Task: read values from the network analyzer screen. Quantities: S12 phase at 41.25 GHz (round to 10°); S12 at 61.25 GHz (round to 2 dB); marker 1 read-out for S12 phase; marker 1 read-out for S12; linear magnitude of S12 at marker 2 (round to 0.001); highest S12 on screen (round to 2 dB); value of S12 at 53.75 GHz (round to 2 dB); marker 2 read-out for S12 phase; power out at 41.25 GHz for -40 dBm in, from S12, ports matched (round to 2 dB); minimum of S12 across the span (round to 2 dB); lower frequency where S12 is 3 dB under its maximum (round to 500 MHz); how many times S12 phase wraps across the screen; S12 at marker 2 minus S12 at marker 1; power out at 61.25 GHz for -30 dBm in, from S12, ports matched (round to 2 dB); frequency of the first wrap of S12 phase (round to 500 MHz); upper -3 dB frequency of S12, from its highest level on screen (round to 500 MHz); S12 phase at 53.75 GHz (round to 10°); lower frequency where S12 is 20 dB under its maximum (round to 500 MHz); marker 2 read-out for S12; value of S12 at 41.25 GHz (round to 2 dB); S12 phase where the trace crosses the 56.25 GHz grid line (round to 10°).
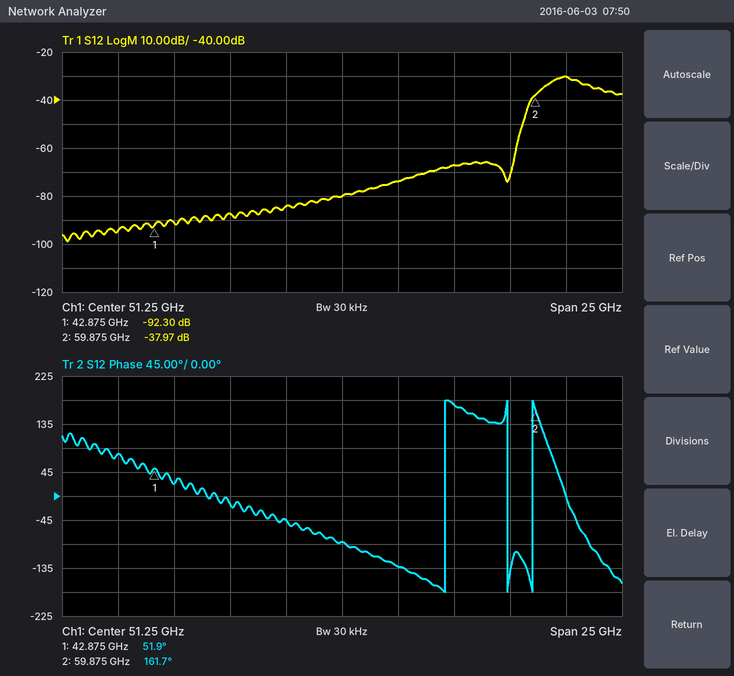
80°
-30 dB
51.9°
-92.30 dB
0.013
-30 dB
-74 dB
161.7°
-134 dBm
-98 dB
60.5 GHz
3
54.33 dB
-60 dBm
56.0 GHz
62.0 GHz
-130°
59.5 GHz
-37.97 dB
-94 dB
170°
